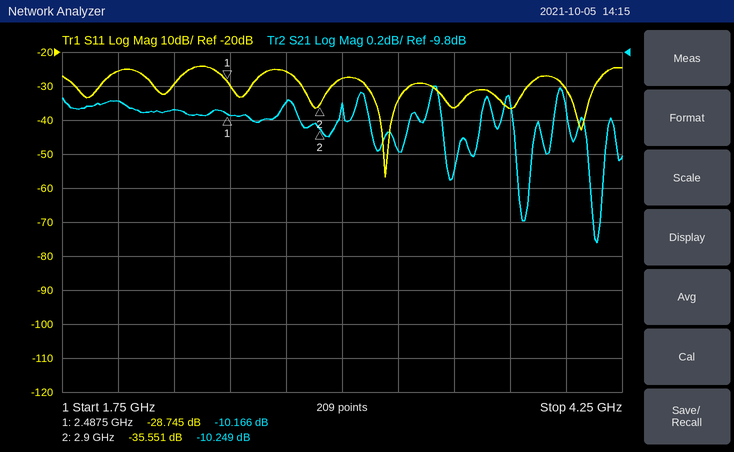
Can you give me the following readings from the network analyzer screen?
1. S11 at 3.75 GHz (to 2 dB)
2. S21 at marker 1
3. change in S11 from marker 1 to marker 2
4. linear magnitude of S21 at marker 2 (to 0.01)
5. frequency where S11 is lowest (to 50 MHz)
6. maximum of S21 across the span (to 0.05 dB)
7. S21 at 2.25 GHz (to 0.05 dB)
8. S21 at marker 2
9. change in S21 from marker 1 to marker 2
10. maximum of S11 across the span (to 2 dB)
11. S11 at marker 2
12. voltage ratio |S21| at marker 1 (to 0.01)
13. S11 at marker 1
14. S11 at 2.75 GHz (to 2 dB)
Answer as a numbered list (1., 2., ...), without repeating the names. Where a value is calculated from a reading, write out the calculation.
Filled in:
1. -36 dB
2. -10.166 dB
3. -35.551 − (-28.745) = -6.806 dB
4. 10^(-10.249/20) ≈ 0.31
5. 3.20 GHz
6. -10.00 dB
7. -10.15 dB
8. -10.249 dB
9. -10.249 − (-10.166) = -0.083 dB
10. -24 dB
11. -35.551 dB
12. 10^(-10.166/20) ≈ 0.31
13. -28.745 dB
14. -26 dB
